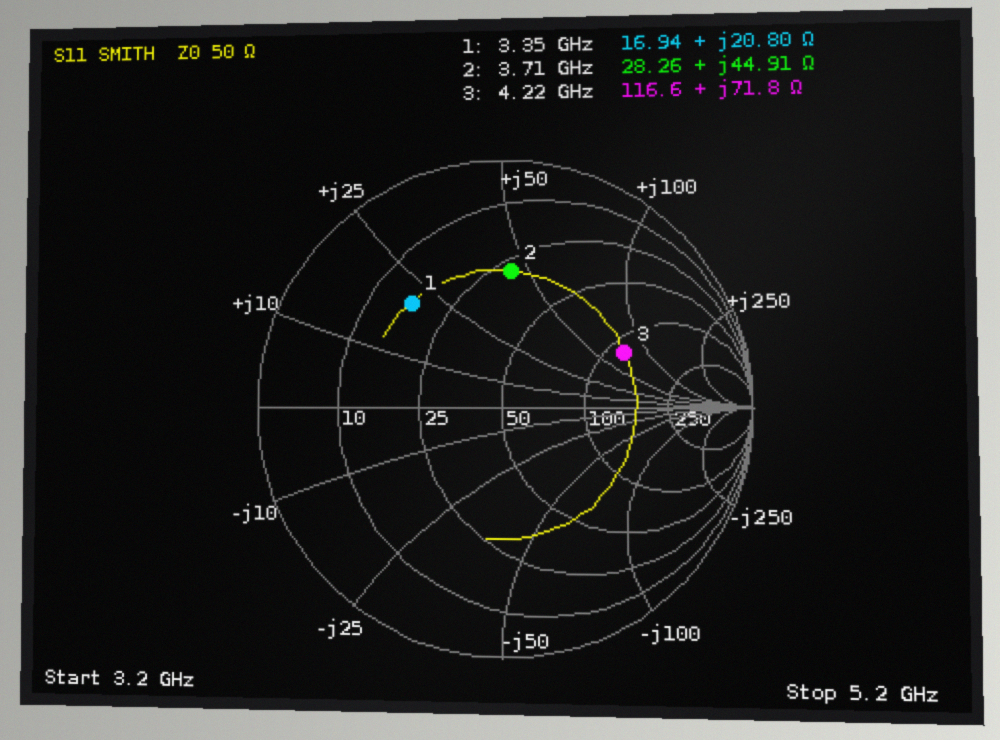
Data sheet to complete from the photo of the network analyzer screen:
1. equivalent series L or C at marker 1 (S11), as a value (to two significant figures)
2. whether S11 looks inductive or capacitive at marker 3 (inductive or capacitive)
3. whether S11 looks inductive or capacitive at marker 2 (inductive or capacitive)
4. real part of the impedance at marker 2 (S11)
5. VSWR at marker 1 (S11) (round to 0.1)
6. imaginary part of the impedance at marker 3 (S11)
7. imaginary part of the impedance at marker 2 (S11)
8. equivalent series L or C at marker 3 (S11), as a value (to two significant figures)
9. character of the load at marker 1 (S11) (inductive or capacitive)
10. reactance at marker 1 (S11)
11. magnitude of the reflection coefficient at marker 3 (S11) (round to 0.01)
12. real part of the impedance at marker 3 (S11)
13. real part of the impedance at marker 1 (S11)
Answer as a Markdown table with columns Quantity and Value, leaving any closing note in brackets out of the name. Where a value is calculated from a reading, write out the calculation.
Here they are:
| Quantity | Value |
|---|---|
| equivalent series L or C at marker 1 (S11), as a value | L = 20.8 Ω/(2π × 3.35 GHz) ≈ 988 pH, so 990 pH to two significant figures |
| whether S11 looks inductive or capacitive at marker 3 | inductive |
| whether S11 looks inductive or capacitive at marker 2 | inductive |
| real part of the impedance at marker 2 | 28.26 Ω |
| VSWR at marker 1 (S11) | 3.5 |
| imaginary part of the impedance at marker 3 | +71.8 Ω |
| imaginary part of the impedance at marker 2 | +44.91 Ω |
| equivalent series L or C at marker 3 (S11), as a value | L = 71.8 Ω/(2π × 4.22 GHz) ≈ 2.7 nH |
| character of the load at marker 1 (S11) | inductive |
| reactance at marker 1 | +20.80 Ω |
| magnitude of the reflection coefficient at marker 3 (S11) | 0.54 |
| real part of the impedance at marker 3 | 116.6 Ω |
| real part of the impedance at marker 1 | 16.94 Ω |
